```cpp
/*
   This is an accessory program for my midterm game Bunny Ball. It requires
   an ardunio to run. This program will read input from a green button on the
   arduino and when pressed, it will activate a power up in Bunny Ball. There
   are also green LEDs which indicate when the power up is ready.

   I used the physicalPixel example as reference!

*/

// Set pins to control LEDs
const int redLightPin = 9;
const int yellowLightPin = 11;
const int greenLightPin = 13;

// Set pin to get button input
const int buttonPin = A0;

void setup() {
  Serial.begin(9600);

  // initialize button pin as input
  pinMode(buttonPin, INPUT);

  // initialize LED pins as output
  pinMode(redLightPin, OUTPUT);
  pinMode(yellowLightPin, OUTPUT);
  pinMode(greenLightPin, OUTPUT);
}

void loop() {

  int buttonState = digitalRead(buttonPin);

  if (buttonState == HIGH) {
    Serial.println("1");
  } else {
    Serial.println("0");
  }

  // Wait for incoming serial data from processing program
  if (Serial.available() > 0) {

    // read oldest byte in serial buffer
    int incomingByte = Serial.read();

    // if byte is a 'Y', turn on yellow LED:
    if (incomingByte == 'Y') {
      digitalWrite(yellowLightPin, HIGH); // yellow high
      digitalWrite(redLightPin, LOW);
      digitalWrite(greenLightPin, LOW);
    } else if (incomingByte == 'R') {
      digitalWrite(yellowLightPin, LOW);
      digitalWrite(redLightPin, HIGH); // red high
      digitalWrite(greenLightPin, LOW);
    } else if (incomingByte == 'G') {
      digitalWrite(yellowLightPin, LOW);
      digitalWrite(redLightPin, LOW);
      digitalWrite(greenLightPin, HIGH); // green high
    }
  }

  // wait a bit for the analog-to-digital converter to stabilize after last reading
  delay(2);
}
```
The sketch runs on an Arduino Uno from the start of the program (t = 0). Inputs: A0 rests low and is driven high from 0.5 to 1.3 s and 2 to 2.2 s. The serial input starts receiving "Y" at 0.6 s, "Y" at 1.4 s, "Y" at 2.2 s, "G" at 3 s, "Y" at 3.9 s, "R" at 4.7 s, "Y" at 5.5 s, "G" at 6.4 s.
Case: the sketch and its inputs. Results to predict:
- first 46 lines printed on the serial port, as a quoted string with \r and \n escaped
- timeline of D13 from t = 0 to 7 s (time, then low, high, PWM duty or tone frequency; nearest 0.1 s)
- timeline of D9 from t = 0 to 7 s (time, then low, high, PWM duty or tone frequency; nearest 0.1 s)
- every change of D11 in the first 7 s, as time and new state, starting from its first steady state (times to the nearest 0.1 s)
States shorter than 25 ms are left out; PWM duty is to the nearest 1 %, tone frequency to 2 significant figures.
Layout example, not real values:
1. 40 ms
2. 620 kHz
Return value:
1. "0\r\n0\r\n0\r\n0\r\n0\r\n0\r\n0\r\n0\r\n0\r\n0\r\n0\r\n0\r\n0\r\n0\r\n0\r\n0\r\n0\r\n0\r\n0\r\n0\r\n0\r\n0\r\n0\r\n0\r\n0\r\n0\r\n0\r\n0\r\n0\r\n0\r\n0\r\n0\r\n0\r\n0\r\n0\r\n0\r\n0\r\n0\r\n0\r\n0\r\n0\r\n0\r\n0\r\n0\r\n0\r\n0\r\n"
2. 0 s low; 3 s high; 3.9 s low; 6.4 s high
3. 0 s low; 4.7 s high; 5.5 s low
4. 0 s low; 0.6 s high; 3 s low; 3.9 s high; 4.7 s low; 5.5 s high; 6.4 s low
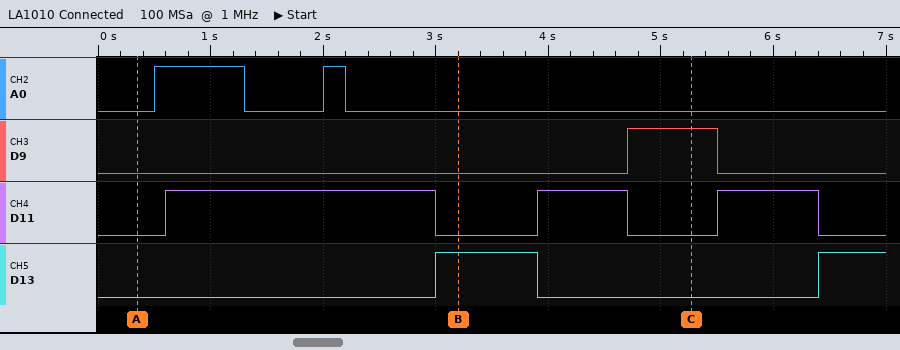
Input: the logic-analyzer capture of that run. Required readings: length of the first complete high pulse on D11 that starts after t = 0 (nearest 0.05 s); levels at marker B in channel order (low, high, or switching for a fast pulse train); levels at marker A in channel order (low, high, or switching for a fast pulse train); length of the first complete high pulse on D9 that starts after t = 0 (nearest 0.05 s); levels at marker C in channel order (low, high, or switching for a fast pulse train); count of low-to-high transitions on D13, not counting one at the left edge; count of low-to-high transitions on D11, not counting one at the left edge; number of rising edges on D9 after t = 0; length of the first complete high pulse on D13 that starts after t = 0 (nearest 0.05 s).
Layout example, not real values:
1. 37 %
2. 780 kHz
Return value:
1. 2.40 s
2. A0 low, D9 low, D11 low, D13 high
3. A0 low, D9 low, D11 low, D13 low
4. 0.80 s
5. A0 low, D9 high, D11 low, D13 low
6. 2
7. 3
8. 1
9. 0.90 s
